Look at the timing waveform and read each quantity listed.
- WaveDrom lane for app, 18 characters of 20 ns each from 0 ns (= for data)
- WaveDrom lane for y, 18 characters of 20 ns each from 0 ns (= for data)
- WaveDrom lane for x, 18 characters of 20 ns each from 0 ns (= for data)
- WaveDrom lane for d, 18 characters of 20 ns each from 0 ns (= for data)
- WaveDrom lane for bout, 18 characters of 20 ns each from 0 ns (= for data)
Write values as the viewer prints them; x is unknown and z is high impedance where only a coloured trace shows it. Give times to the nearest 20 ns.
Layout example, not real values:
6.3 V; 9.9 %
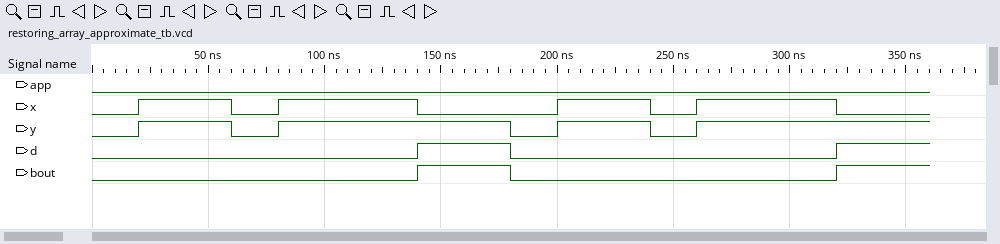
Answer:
{name: 'app', wave: '0.................'}; {name: 'y', wave: '01.01....01.01....'}; {name: 'x', wave: '01.01..0..1.01..0.'}; {name: 'd', wave: '0......1.0......1.'}; {name: 'bout', wave: '0......1.0......1.'}
